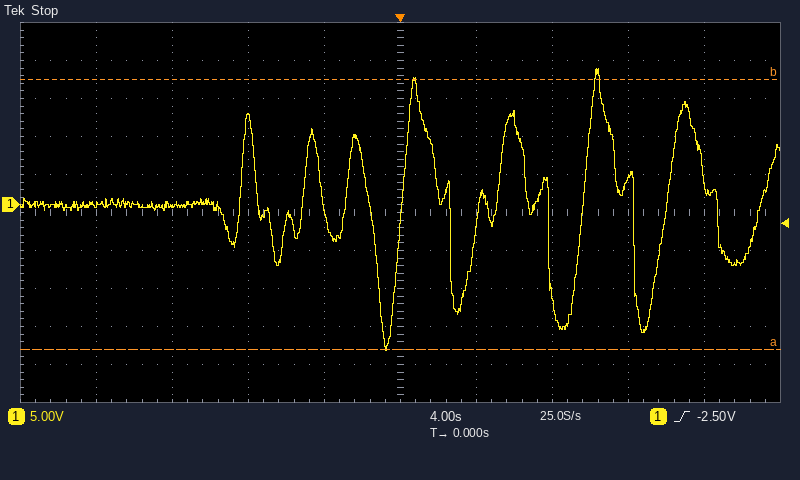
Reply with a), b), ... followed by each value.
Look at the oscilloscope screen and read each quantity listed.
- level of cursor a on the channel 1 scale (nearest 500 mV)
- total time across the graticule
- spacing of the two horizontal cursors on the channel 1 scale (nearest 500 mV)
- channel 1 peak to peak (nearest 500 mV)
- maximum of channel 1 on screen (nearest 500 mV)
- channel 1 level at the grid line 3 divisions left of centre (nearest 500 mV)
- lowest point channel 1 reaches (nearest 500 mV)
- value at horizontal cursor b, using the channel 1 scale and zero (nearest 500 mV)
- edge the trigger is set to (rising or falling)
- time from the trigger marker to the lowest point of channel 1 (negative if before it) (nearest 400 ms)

a) -19.0 V
b) 40 s
c) 35.5 V
d) 37.0 V
e) 18.0 V
f) 0.0 V
g) -19.0 V
h) 16.5 V
i) rising
j) -800 ms
